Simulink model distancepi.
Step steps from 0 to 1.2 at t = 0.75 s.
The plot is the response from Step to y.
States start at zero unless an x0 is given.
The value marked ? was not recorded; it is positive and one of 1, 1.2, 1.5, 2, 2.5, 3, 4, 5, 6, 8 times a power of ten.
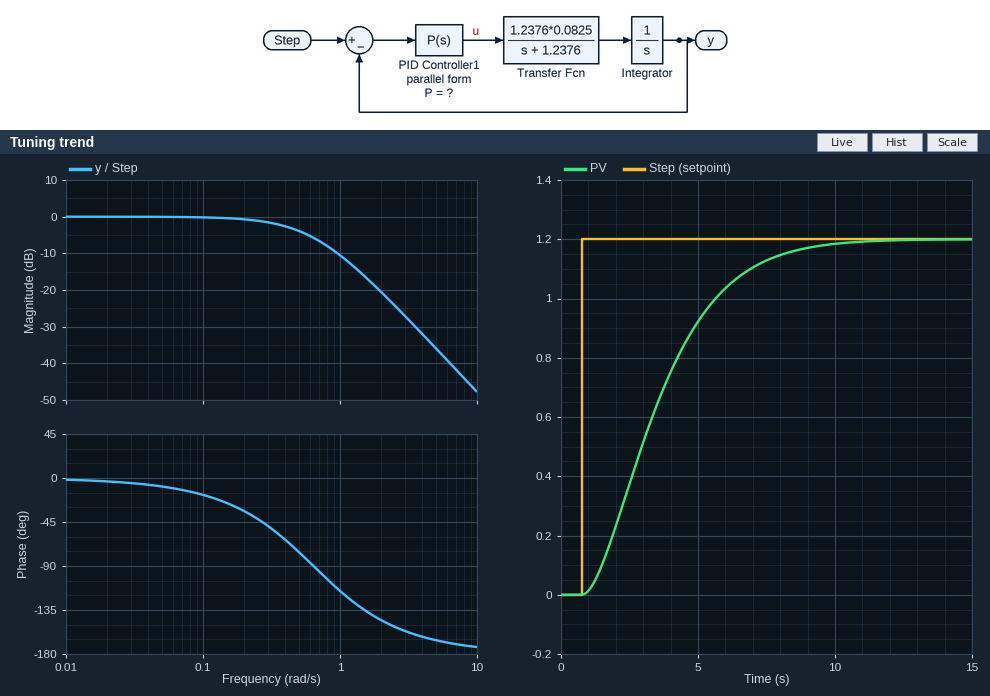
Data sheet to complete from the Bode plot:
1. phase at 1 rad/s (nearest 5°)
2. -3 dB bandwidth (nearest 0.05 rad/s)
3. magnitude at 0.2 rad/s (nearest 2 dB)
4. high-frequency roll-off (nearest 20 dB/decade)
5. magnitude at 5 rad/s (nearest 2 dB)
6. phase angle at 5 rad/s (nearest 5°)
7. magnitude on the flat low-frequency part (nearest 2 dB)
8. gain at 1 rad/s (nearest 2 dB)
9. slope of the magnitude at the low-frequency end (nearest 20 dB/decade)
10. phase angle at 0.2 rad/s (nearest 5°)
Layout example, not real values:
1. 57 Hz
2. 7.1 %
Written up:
1. -115°
2. 0.45 rad/s
3. 0 dB
4. -40 dB/decade
5. -36 dB
6. -165°
7. 0 dB
8. -10 dB
9. 0 dB/decade
10. -35°
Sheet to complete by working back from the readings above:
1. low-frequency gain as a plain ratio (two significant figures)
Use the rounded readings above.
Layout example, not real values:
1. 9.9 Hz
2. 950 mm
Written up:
1. 1.0
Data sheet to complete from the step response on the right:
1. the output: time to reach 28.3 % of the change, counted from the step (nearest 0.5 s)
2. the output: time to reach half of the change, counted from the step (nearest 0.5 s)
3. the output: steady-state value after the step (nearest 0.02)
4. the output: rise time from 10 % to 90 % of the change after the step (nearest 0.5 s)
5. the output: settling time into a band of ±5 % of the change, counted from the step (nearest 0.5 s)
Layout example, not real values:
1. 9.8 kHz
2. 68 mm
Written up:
1. 1.5 s
2. 2.5 s
3. 1.20
4. 5.0 s
5. 7.0 s
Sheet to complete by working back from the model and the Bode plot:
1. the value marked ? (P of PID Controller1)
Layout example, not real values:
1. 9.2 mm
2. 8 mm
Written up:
1. 4
